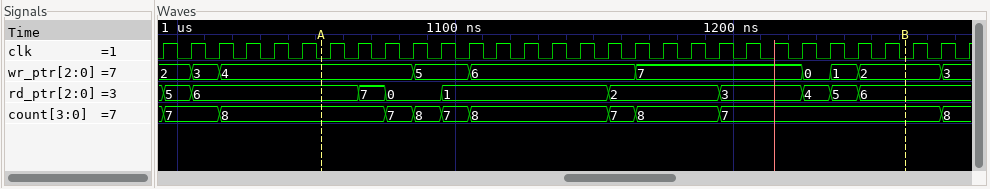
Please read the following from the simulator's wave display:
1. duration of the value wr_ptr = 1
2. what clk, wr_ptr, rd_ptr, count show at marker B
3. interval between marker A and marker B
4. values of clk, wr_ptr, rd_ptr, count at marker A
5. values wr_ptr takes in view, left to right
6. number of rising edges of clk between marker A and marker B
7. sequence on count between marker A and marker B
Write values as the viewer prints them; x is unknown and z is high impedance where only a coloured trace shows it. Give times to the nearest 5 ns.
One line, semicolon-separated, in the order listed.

10 ns; clk=0, wr_ptr=2, rd_ptr=6, count=7; 210 ns; clk=0, wr_ptr=4, rd_ptr=6, count=8; 2, 3, 4, 5, 6, 7, 0, 1, 2, 3; 21; 8, 7, 8, 7, 8, 7, 8, 7
